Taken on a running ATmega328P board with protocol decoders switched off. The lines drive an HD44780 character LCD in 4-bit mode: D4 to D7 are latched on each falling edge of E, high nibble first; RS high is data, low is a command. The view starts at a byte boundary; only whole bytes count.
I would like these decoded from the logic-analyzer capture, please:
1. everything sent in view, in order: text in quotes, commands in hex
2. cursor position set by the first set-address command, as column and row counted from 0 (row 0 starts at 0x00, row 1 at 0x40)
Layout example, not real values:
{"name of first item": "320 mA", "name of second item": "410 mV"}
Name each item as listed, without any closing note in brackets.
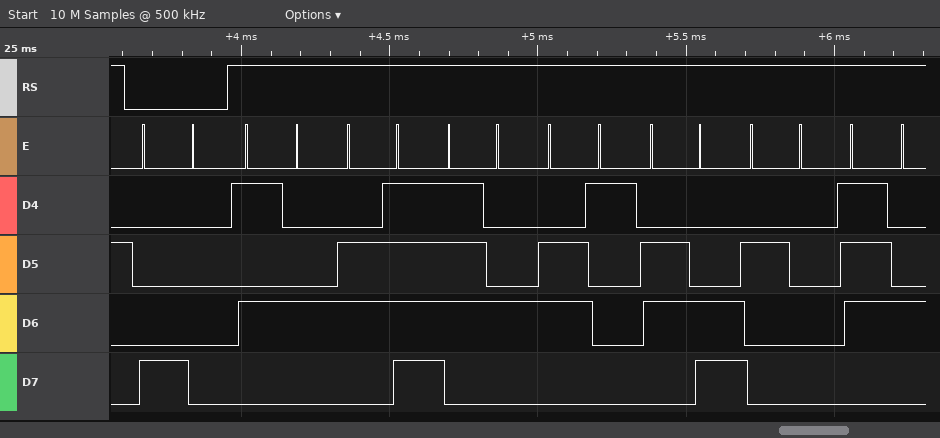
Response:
{"everything sent in view, in order: text in quotes, commands in hex": "0x80 \"Total t\"", "cursor position set by the first set-address command, as column and row counted from 0": "column 0, row 0"}
